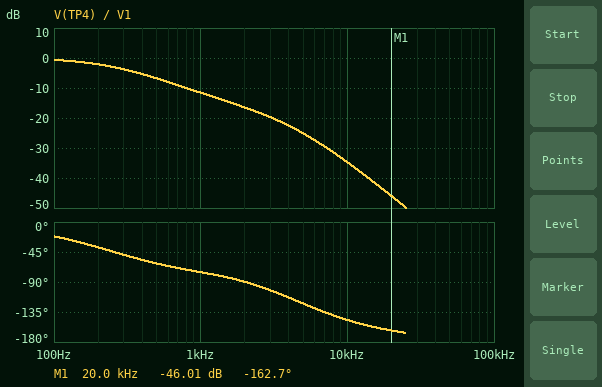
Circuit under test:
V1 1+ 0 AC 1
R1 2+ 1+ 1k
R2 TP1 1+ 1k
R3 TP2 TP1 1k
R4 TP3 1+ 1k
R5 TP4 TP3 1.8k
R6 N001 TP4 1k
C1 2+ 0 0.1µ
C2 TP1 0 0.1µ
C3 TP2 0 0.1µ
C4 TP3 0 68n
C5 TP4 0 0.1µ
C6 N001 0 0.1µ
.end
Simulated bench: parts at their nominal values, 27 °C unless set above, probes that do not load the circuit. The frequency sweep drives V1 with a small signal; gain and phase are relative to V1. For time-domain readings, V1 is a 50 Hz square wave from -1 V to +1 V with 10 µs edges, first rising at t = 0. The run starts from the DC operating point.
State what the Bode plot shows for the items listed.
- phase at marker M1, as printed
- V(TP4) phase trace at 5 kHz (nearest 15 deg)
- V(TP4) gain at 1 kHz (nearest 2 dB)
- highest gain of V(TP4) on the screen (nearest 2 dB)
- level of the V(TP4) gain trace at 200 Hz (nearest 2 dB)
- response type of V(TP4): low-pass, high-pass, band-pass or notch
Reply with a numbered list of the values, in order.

1. -162.7 deg
2. -120 deg
3. -12 dB
4. 0 dB
5. -2 dB
6. low-pass
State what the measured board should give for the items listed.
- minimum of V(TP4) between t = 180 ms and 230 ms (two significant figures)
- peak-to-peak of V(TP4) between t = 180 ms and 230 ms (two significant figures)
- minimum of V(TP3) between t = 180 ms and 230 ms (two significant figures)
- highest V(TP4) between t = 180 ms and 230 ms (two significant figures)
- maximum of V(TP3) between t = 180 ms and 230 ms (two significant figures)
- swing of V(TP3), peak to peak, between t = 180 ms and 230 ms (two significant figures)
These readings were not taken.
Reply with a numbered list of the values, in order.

1. -1.0 V
2. 2.0 V
3. -1.0 V
4. 1.0 V
5. 1.0 V
6. 2.0 V
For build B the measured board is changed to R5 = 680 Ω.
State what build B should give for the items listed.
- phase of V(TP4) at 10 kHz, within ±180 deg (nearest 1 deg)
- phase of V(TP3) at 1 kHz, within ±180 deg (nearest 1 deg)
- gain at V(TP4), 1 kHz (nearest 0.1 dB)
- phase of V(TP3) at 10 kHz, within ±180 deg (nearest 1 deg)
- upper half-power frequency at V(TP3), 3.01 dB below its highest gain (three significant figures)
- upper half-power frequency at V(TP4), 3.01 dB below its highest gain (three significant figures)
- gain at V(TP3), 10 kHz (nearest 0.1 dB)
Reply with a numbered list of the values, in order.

1. -132 deg
2. -32 deg
3. -8.3 dB
4. -63 deg
5. 482 Hz
6. 384 Hz
7. -14.2 dB
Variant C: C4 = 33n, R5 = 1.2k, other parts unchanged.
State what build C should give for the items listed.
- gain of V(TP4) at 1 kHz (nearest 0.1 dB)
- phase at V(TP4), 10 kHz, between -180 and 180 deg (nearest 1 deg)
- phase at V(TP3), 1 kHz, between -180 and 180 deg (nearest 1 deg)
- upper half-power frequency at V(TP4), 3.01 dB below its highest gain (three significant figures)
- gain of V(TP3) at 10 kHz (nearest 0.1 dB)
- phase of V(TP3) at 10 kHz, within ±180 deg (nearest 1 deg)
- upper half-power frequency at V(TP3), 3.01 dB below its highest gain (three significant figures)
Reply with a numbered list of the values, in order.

1. -9.5 dB
2. -125 deg
3. -19 deg
4. 322 Hz
5. -9.0 dB
6. -50 deg
7. 552 Hz
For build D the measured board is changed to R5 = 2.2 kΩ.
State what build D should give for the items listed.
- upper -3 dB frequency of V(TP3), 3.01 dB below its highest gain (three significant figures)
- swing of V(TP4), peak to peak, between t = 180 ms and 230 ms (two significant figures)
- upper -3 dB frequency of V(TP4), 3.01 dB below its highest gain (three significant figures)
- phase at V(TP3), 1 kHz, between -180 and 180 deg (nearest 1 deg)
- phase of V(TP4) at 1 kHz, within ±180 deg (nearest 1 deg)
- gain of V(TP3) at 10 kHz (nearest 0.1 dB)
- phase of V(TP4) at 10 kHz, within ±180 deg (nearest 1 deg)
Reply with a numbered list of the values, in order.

1. 722 Hz
2. 2.0 V
3. 225 Hz
4. -22 deg
5. -78 deg
6. -13.1 dB
7. -149 deg
